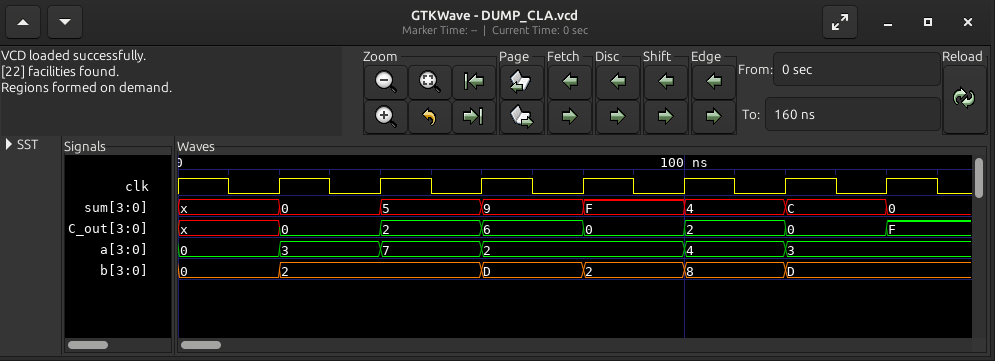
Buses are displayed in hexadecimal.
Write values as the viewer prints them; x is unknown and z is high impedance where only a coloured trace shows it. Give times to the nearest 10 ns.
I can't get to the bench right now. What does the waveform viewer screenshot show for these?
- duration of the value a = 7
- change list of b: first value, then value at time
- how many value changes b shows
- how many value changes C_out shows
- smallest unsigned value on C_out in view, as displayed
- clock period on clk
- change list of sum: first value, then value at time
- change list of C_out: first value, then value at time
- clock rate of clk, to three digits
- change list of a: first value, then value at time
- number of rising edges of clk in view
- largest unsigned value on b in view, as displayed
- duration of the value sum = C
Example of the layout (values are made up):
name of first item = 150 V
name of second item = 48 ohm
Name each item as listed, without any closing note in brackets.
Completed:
duration of the value a = 7 = 20 ns
change list of b: first value, then value at time = 0, 2 at 20 ns, D at 60 ns, 2 at 80 ns, 8 at 100 ns, D at 120 ns
how many value changes b shows = 5
how many value changes C_out shows = 7
smallest unsigned value on C_out in view, as displayed = 0
clock period on clk = 20 ns
change list of sum: first value, then value at time = x, 0 at 20 ns, 5 at 40 ns, 9 at 60 ns, F at 80 ns, 4 at 100 ns, C at 120 ns, 0 at 140 ns
change list of C_out: first value, then value at time = x, 0 at 20 ns, 2 at 40 ns, 6 at 60 ns, 0 at 80 ns, 2 at 100 ns, 0 at 120 ns, F at 140 ns
clock rate of clk, to three digits = 50.0 MHz
change list of a: first value, then value at time = 0, 3 at 20 ns, 7 at 40 ns, 2 at 60 ns, 4 at 100 ns, 3 at 120 ns
number of rising edges of clk in view = 7
largest unsigned value on b in view, as displayed = D
duration of the value sum = C = 20 ns
